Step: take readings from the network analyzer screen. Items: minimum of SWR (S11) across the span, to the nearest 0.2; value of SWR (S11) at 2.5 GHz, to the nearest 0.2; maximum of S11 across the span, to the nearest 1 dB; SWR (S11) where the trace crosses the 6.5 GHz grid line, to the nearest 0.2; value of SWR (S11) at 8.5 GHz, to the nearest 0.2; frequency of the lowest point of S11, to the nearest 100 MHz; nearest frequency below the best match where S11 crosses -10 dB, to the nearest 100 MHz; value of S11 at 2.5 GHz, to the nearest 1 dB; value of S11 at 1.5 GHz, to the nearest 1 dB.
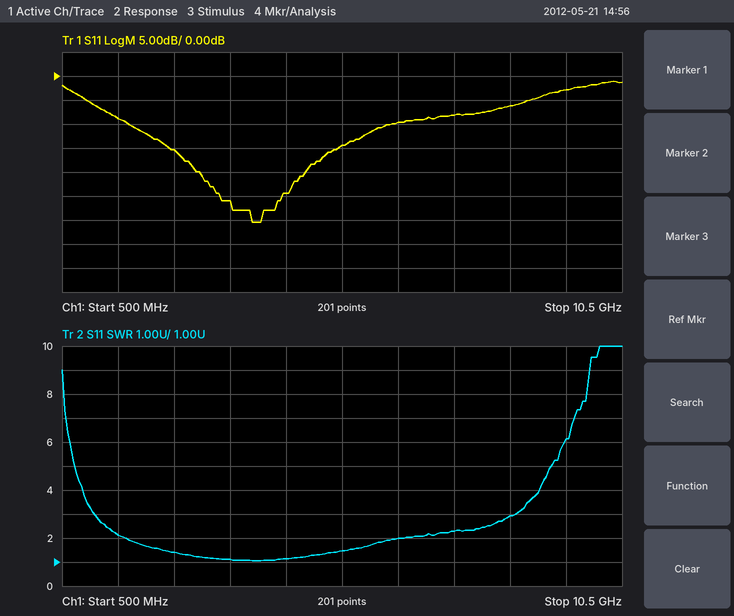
1.0
1.4
-1 dB
2.0
3.0
3.9 GHz
1.7 GHz
-15 dB
-9 dB
